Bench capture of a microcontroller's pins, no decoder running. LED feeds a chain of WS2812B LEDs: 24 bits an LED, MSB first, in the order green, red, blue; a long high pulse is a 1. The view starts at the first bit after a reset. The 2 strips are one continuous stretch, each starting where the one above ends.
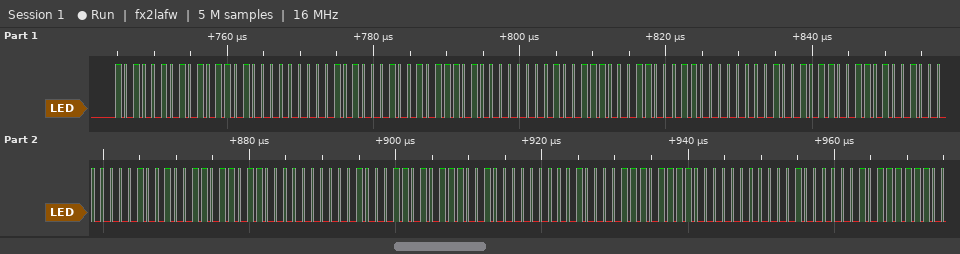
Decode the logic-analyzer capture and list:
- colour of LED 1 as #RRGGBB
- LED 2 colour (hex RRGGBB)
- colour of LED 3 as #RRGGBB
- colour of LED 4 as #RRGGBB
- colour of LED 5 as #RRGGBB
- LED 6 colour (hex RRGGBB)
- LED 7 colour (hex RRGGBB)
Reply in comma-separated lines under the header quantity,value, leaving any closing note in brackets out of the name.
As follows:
quantity,value
colour of LED 1 as #RRGGBB,#5AA500
LED 2 colour,#5DA200
colour of LED 3 as #RRGGBB,#639C00
colour of LED 4 as #RRGGBB,#699600
colour of LED 5 as #RRGGBB,#6C9300
LED 6 colour,#728D00
LED 7 colour,#788700
